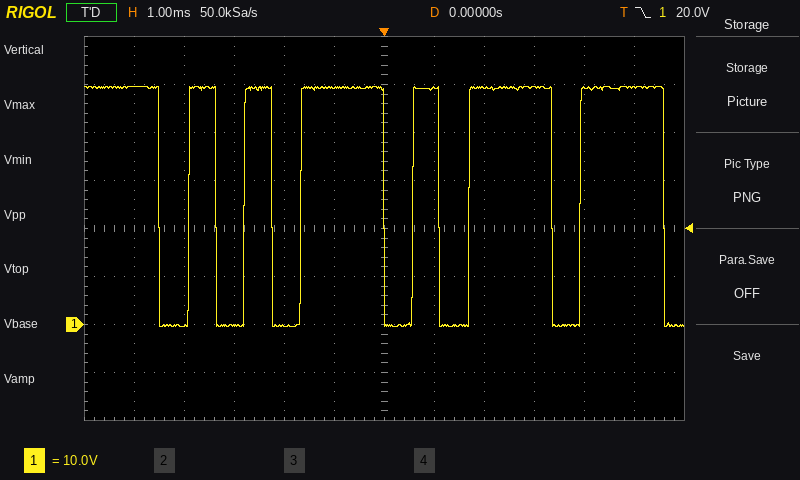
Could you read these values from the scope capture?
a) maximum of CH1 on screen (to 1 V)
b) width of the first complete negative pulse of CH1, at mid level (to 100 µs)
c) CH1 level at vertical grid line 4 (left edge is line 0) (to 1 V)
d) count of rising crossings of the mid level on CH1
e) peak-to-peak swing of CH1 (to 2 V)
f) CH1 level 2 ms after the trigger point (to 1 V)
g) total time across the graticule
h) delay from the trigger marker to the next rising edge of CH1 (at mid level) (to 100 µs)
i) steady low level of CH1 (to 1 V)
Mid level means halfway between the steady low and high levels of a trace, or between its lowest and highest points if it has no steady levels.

50 V
600 µs
0 V
6
50 V
49 V
12 ms
600 µs
0 V
